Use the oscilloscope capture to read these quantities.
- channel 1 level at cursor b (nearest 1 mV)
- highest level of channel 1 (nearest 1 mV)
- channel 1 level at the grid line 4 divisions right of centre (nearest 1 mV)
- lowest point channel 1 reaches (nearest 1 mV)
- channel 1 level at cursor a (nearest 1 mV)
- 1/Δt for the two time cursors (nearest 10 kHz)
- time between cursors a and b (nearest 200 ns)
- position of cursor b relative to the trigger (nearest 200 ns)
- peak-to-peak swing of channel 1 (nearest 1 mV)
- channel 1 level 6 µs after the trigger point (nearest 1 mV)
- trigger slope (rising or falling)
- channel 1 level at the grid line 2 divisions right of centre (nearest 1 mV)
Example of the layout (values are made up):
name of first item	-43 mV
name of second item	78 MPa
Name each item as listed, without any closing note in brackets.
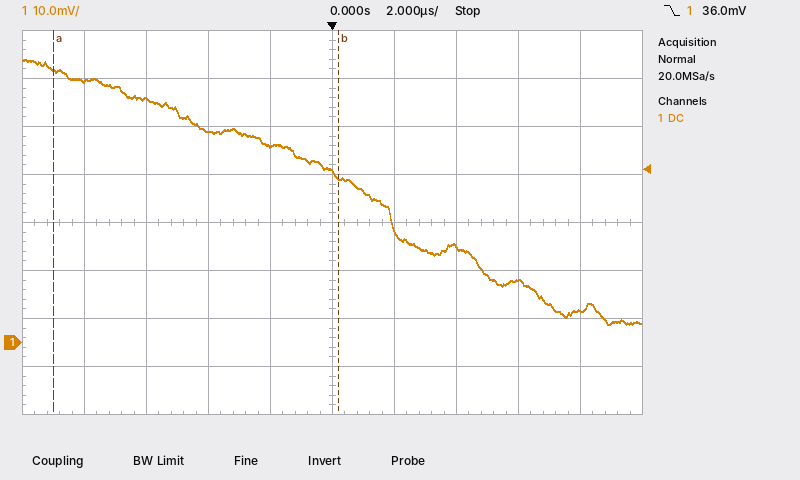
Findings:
channel 1 level at cursor b	34 mV
highest level of channel 1	59 mV
channel 1 level at the grid line 4 divisions right of centre	7 mV
lowest point channel 1 reaches	4 mV
channel 1 level at cursor a	57 mV
1/Δt for the two time cursors	110 kHz
time between cursors a and b	9.2 µs
position of cursor b relative to the trigger	+200 ns
peak-to-peak swing of channel 1	55 mV
channel 1 level 6 µs after the trigger point	13 mV
trigger slope	falling
channel 1 level at the grid line 2 divisions right of centre	20 mV
